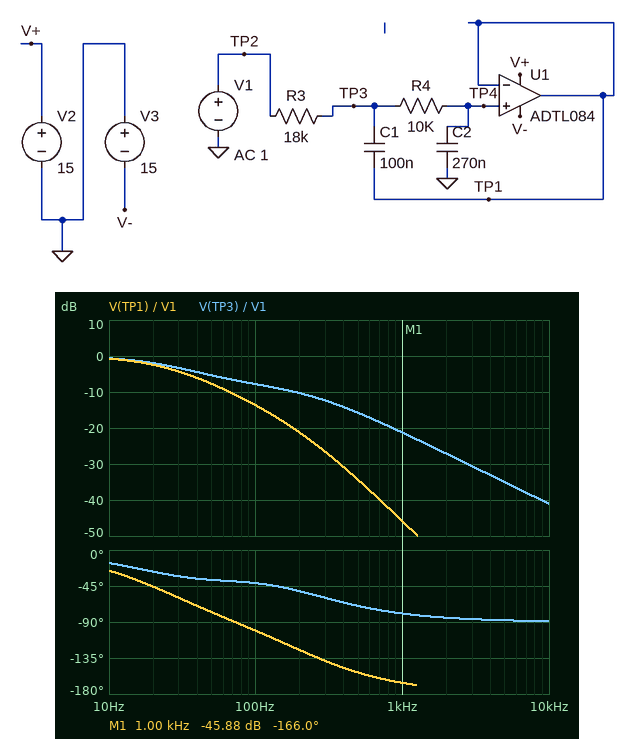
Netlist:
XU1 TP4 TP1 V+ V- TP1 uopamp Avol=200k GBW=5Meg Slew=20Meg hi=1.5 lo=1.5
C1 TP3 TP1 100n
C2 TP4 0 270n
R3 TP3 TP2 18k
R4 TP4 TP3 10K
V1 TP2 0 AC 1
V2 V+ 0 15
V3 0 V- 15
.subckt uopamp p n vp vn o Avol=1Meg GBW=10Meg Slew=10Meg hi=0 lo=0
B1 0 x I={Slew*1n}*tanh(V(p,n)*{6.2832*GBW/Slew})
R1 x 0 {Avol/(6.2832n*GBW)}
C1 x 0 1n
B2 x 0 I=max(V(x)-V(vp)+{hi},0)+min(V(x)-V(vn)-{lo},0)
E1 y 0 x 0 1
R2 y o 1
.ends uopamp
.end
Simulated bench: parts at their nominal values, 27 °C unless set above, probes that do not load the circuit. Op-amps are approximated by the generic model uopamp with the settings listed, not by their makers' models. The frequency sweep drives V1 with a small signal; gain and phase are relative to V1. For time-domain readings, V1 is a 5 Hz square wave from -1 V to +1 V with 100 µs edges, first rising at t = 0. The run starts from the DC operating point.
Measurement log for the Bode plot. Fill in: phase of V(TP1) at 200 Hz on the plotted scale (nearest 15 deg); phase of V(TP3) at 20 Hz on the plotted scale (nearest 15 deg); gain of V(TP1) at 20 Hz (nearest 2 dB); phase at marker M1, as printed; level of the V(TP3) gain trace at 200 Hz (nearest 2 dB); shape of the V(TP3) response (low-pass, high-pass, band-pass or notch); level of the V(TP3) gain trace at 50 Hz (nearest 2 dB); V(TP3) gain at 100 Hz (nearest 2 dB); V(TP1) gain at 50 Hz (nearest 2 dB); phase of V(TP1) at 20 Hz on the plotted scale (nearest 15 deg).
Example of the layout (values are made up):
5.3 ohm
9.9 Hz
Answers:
-120 deg
-30 deg
-2 dB
-166.0 deg
-10 dB
low-pass
-6 dB
-8 dB
-8 dB
-45 deg
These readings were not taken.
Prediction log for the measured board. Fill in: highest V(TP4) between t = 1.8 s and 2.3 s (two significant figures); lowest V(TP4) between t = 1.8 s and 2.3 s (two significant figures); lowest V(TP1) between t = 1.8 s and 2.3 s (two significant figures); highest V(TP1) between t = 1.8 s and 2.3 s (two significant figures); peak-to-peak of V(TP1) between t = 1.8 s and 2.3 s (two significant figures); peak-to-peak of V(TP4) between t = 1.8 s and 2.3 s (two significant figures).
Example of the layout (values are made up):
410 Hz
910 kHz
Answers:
1.0 V
-1.0 V
-1.0 V
1.0 V
2.0 V
2.0 V
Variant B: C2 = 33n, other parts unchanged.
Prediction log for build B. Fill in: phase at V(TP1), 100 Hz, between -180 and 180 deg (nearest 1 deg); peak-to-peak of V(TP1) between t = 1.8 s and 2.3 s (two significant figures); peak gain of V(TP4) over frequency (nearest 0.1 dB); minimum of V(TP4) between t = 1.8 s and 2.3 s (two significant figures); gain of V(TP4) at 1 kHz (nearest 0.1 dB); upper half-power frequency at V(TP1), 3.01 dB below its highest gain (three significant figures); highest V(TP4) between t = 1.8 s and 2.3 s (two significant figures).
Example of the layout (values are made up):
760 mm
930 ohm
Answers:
-37 deg
2.4 V
0.4 dB
-1.2 V
-27.3 dB
230 Hz
1.2 V
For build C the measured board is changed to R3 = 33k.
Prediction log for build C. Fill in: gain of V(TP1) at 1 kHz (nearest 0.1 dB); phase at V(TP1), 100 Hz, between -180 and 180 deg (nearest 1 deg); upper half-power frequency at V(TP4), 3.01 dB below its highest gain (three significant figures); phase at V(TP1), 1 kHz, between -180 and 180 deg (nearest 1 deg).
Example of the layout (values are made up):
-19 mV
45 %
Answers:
-51.1 dB
-109 deg
14.7 Hz
-168 deg
